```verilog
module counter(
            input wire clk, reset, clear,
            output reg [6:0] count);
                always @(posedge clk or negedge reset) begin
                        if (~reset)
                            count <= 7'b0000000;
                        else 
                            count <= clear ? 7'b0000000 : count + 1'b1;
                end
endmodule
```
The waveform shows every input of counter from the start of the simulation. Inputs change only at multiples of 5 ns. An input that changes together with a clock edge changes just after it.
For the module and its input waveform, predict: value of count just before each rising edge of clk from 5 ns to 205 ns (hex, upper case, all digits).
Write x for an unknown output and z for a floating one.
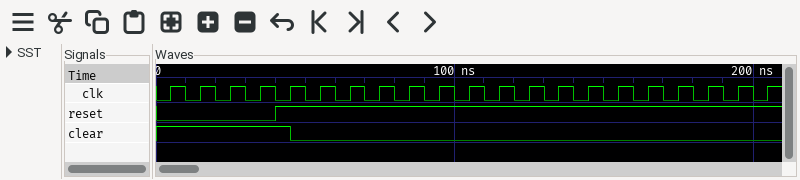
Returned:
00, 00, 00, 00, 00, 00, 01, 02, 03, 04, 05, 06, 07, 08, 09, 0A, 0B, 0C, 0D, 0E, 0F
